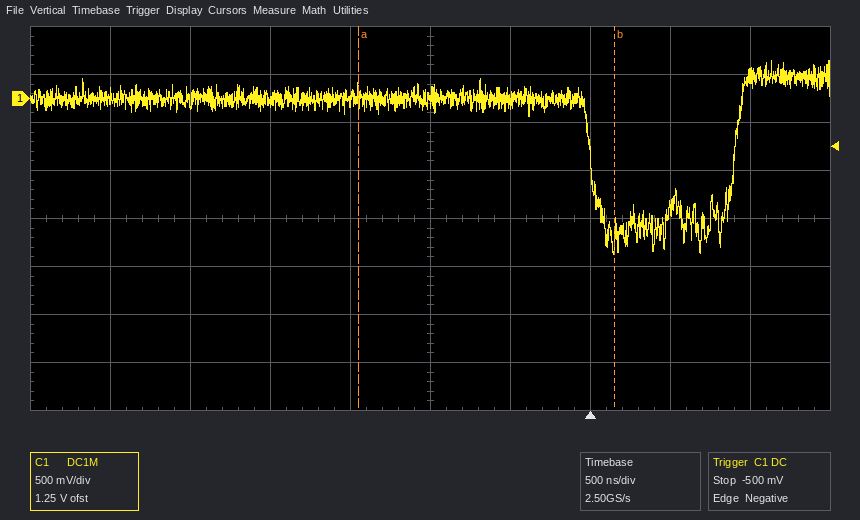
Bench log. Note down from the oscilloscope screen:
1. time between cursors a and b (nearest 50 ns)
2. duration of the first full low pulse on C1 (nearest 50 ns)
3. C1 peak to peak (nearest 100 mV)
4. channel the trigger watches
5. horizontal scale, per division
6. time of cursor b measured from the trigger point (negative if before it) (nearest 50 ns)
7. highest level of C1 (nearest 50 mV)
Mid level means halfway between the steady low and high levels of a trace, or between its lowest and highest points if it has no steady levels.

1.60 µs
900 ns
2.00 V
C1
500 ns
+150 ns
400 mV
